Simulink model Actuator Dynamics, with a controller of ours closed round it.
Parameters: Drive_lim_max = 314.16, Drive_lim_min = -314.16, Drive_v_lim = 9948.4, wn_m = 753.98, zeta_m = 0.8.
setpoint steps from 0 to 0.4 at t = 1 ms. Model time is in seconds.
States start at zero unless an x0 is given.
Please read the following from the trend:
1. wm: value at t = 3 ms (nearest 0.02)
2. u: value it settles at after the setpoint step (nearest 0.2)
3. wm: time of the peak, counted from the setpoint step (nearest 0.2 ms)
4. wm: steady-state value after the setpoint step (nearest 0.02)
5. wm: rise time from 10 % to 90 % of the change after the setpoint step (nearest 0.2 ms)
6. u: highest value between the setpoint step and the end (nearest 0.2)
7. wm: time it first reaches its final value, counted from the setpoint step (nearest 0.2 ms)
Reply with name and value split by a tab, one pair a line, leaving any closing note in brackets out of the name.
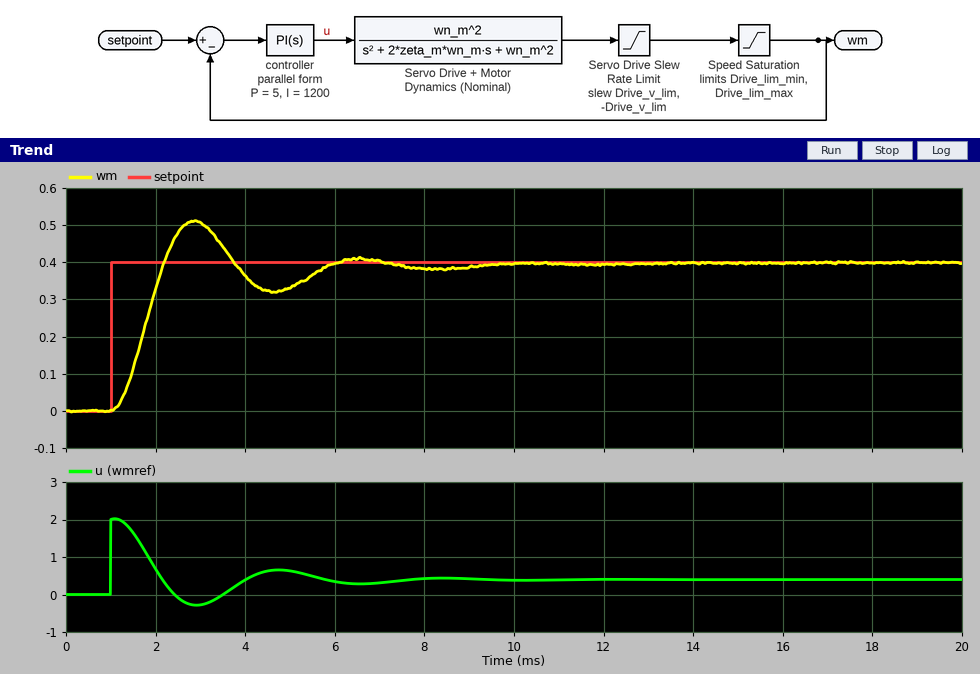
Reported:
wm: value at t = 3 ms	0.50
u: value it settles at after the setpoint step	0.4
wm: time of the peak, counted from the setpoint step	1.8 ms
wm: steady-state value after the setpoint step	0.40
wm: rise time from 10 % to 90 % of the change after the setpoint step	0.8 ms
u: highest value between the setpoint step and the end	2.0
wm: time it first reaches its final value, counted from the setpoint step	1.2 ms
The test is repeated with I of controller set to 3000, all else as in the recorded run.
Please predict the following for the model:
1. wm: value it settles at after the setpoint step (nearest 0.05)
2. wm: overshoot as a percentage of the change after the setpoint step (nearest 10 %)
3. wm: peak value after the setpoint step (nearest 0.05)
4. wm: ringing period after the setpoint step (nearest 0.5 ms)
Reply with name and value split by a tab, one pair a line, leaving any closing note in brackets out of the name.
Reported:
wm: value it settles at after the setpoint step	0.40
wm: overshoot as a percentage of the change after the setpoint step	50 %
wm: peak value after the setpoint step	0.60
wm: ringing period after the setpoint step	3.5 ms
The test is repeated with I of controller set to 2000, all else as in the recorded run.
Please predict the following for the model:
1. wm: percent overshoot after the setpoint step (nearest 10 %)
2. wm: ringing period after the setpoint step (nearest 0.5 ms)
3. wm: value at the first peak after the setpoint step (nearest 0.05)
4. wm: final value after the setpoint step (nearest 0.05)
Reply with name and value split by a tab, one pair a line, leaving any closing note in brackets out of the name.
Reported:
wm: percent overshoot after the setpoint step	40 %
wm: ringing period after the setpoint step	3.5 ms
wm: value at the first peak after the setpoint step	0.55
wm: final value after the setpoint step	0.40
